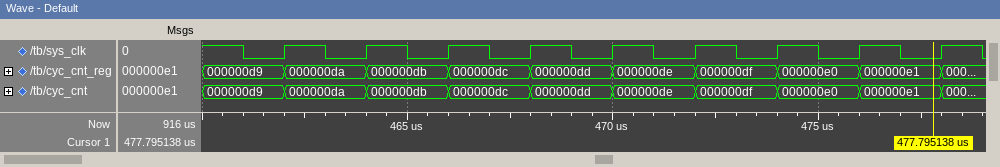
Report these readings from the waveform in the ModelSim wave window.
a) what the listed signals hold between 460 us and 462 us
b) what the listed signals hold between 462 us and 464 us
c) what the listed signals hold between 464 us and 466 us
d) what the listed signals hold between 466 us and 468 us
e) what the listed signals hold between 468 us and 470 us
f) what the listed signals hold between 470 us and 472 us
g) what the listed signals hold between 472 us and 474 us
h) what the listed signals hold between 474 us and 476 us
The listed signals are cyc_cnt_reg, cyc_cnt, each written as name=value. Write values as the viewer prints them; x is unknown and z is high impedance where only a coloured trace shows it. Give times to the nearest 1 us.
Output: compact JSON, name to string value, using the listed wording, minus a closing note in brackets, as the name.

{"what the listed signals hold between 460 us and 462 us": "cyc_cnt_reg=000000d9, cyc_cnt=000000d9", "what the listed signals hold between 462 us and 464 us": "cyc_cnt_reg=000000da, cyc_cnt=000000da", "what the listed signals hold between 464 us and 466 us": "cyc_cnt_reg=000000db, cyc_cnt=000000db", "what the listed signals hold between 466 us and 468 us": "cyc_cnt_reg=000000dc, cyc_cnt=000000dc", "what the listed signals hold between 468 us and 470 us": "cyc_cnt_reg=000000dd, cyc_cnt=000000dd", "what the listed signals hold between 470 us and 472 us": "cyc_cnt_reg=000000de, cyc_cnt=000000de", "what the listed signals hold between 472 us and 474 us": "cyc_cnt_reg=000000df, cyc_cnt=000000df", "what the listed signals hold between 474 us and 476 us": "cyc_cnt_reg=000000e0, cyc_cnt=000000e0"}
